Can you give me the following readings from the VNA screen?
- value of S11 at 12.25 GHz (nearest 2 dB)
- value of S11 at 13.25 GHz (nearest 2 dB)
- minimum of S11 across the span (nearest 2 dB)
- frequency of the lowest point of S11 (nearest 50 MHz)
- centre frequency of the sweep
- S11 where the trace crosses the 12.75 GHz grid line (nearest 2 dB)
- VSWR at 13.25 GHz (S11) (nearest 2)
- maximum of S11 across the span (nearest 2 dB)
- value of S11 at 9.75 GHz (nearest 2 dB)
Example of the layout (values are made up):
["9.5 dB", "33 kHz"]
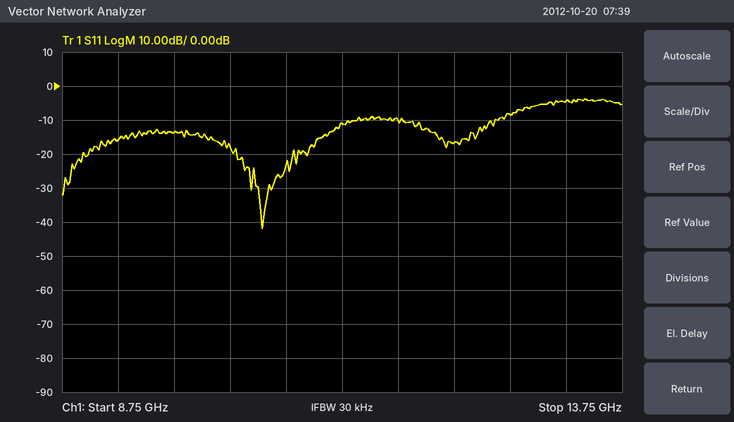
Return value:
["-16 dB", "-4 dB", "-42 dB", "10.55 GHz", "11.25 GHz", "-8 dB", "4", "-4 dB", "-14 dB"]
